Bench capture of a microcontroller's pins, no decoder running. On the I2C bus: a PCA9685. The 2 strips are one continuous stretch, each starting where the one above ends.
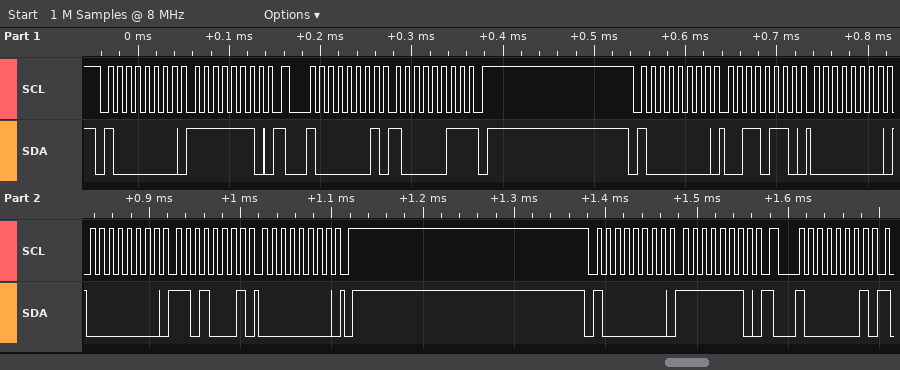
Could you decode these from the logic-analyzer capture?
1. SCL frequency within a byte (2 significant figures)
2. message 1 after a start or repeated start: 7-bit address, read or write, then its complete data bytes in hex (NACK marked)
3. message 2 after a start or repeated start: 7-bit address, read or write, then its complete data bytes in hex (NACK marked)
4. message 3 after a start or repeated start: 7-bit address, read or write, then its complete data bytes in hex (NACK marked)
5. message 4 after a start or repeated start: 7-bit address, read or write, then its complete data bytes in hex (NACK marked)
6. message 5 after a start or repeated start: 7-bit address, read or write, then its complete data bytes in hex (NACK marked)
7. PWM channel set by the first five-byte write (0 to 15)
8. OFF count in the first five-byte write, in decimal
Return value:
100 kHz
0x40 write: FE
0x40 read: 83 NACK
0x40 write: 36 00 00 D1 00
0x40 write: FE
0x40 read
12
209
